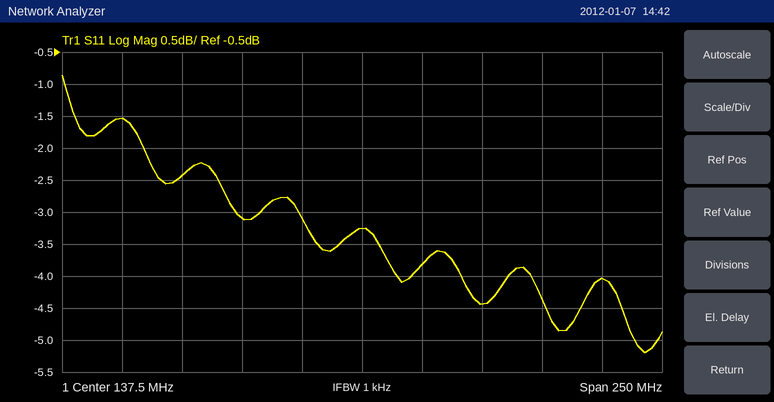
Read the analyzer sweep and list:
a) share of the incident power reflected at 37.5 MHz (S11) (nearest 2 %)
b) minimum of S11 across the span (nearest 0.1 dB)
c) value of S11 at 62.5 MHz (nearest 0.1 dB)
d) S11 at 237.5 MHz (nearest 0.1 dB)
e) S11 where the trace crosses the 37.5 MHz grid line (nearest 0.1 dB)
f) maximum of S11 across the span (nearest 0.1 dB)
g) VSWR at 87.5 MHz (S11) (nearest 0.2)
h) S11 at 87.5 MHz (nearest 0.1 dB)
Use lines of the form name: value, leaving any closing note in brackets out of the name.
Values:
share of the incident power reflected at 37.5 MHz (S11): 70 %
minimum of S11 across the span: -5.2 dB
value of S11 at 62.5 MHz: -2.4 dB
S11 at 237.5 MHz: -4.0 dB
S11 where the trace crosses the 37.5 MHz grid line: -1.5 dB
maximum of S11 across the span: -0.9 dB
VSWR at 87.5 MHz (S11): 5.6
S11 at 87.5 MHz: -3.1 dB
